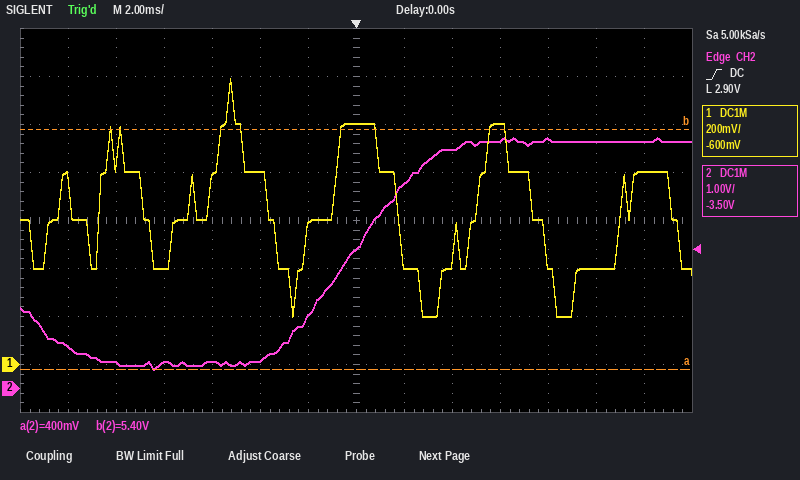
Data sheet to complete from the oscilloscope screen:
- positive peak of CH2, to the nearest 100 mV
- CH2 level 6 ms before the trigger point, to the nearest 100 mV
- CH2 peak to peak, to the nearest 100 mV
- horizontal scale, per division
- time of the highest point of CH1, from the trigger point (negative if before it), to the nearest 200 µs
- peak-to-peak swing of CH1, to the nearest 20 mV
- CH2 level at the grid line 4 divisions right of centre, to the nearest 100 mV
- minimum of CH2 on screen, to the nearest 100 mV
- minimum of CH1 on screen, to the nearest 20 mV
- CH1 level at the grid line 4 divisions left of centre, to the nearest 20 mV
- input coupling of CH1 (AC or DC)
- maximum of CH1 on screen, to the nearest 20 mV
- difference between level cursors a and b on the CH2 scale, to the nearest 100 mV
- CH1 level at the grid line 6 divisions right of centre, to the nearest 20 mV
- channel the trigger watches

5.2 V
600 mV
4.8 V
2 ms
-5.2 ms
1.00 V
5.2 V
400 mV
200 mV
400 mV
DC
1.20 V
5.0 V
800 mV
CH2
